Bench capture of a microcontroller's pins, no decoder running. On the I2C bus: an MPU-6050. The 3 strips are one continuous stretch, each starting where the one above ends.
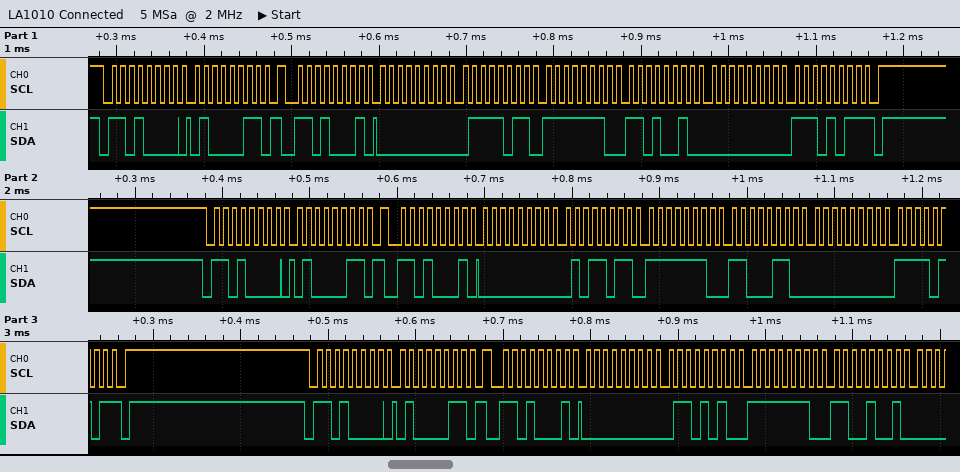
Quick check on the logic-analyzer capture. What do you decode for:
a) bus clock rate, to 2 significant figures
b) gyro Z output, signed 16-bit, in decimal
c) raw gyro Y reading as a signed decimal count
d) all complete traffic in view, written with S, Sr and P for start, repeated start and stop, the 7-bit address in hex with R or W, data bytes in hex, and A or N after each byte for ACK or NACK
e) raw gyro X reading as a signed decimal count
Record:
100 kHz
235
-302
S 68W A 43 A Sr 68R A 00 A 7B A FE A D2 A 00 A EB N P S 68W A 43 A Sr 68R A 00 A 5B A FE A C6 A 00 A F5 N P S 68W A 43 A Sr 68R A 00 A 6A A FE A C9 A
123
